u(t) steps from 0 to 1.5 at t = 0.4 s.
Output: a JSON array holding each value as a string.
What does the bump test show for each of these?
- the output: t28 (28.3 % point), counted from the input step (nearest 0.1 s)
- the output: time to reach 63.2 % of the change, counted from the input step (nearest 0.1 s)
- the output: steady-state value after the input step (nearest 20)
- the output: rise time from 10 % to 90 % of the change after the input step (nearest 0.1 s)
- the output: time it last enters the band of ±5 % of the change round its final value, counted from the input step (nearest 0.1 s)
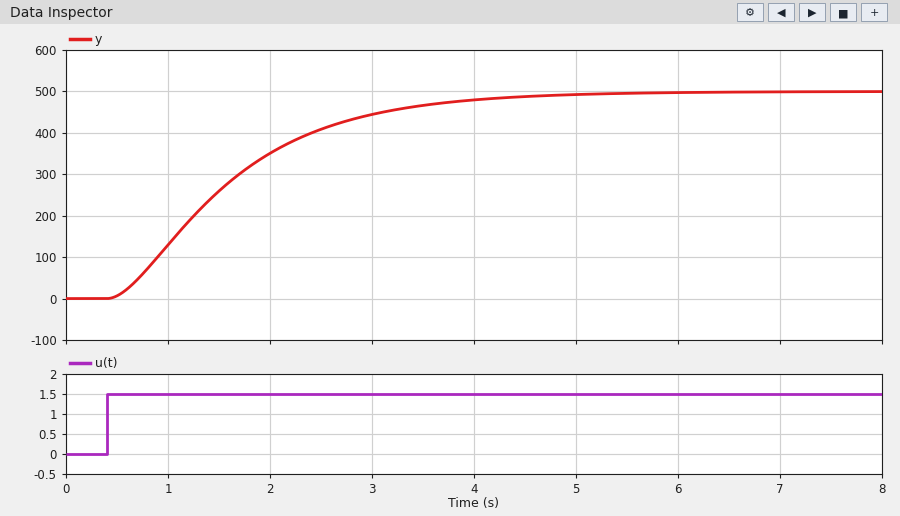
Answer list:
["0.6 s", "1.4 s", "500", "2.4 s", "3.4 s"]
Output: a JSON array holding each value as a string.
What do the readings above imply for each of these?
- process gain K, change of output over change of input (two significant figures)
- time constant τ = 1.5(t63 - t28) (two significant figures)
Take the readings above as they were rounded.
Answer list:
["330", "1.2 s"]
